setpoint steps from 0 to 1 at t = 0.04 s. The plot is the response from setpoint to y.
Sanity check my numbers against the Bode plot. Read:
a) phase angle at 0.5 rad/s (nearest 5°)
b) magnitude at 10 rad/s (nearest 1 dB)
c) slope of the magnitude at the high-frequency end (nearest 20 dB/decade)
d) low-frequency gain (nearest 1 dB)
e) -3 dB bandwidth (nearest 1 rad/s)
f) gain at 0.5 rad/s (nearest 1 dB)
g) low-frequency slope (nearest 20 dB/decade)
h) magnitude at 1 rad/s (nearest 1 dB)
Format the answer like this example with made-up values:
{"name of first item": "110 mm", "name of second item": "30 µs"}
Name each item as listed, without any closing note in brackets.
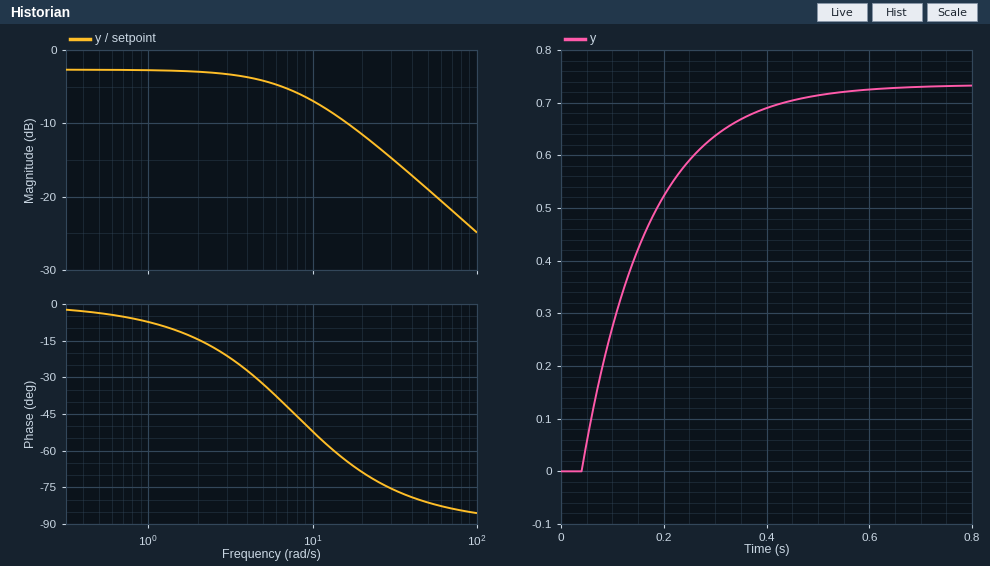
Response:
{"phase angle at 0.5 rad/s": "-5°", "magnitude at 10 rad/s": "-7 dB", "slope of the magnitude at the high-frequency end": "-20 dB/decade", "low-frequency gain": "-3 dB", "-3 dB bandwidth": "8 rad/s", "gain at 0.5 rad/s": "-3 dB", "low-frequency slope": "0 dB/decade", "magnitude at 1 rad/s": "-3 dB"}
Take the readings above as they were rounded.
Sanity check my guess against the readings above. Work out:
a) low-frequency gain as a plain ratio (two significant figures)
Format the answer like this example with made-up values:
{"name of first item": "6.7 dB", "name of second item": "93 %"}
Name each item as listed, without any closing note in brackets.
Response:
{"low-frequency gain as a plain ratio": "0.71"}
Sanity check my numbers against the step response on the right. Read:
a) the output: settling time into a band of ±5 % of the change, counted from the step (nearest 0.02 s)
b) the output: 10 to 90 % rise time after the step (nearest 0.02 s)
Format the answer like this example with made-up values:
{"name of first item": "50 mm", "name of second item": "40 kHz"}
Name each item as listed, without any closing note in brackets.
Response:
{"the output: settling time into a band of ±5 % of the change, counted from the step": "0.38 s", "the output: 10 to 90 % rise time after the step": "0.28 s"}
